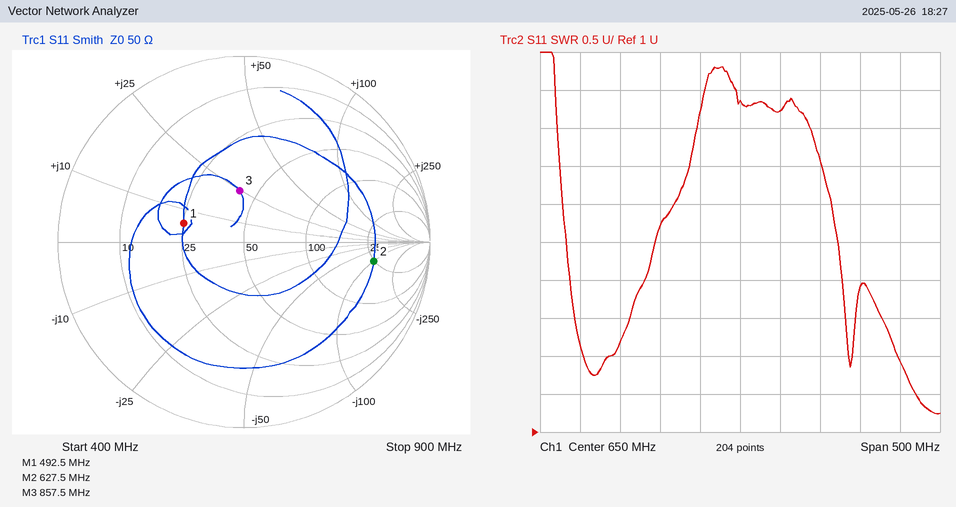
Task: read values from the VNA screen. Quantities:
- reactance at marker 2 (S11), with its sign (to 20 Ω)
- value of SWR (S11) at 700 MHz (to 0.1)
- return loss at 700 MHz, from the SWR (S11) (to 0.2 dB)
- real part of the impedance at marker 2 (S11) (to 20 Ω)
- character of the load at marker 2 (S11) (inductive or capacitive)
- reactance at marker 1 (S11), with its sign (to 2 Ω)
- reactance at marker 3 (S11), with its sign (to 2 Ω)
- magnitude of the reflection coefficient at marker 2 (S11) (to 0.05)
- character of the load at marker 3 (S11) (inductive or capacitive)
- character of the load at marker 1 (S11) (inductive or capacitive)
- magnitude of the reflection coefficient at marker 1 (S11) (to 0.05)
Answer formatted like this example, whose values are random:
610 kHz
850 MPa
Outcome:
-100 Ω
5.2
3.4 dB
240 Ω
capacitive
+6 Ω
+24 Ω
0.70
inductive
inductive
0.35
